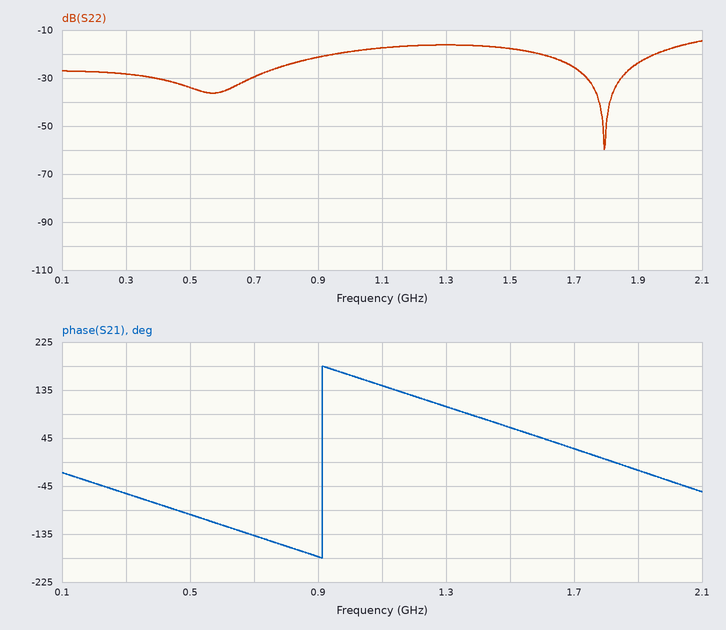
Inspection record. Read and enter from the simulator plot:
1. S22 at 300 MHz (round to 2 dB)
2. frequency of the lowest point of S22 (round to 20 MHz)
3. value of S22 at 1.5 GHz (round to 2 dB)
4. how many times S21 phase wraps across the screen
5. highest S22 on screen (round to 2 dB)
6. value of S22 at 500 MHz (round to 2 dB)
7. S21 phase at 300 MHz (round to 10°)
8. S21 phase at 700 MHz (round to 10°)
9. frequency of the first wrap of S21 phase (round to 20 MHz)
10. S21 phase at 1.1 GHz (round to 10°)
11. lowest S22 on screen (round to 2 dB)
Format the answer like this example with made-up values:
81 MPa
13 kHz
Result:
-28 dB
1.80 GHz
-18 dB
1
-14 dB
-34 dB
-60°
-140°
920 MHz
140°
-60 dB
